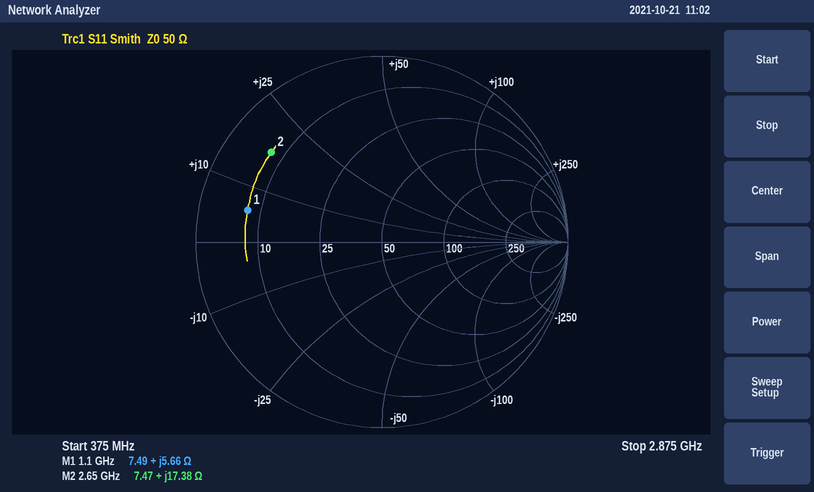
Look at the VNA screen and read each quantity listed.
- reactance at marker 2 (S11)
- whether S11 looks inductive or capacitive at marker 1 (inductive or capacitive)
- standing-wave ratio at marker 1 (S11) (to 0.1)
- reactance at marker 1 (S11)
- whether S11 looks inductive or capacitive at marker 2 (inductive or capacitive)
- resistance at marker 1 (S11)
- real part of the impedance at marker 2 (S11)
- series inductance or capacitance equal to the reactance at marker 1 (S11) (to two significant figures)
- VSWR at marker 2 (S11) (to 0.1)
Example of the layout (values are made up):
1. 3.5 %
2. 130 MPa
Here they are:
1. +17.38 Ω
2. inductive
3. 6.8
4. +5.66 Ω
5. inductive
6. 7.49 Ω
7. 7.47 Ω
8. 820 pH
9. 7.5
